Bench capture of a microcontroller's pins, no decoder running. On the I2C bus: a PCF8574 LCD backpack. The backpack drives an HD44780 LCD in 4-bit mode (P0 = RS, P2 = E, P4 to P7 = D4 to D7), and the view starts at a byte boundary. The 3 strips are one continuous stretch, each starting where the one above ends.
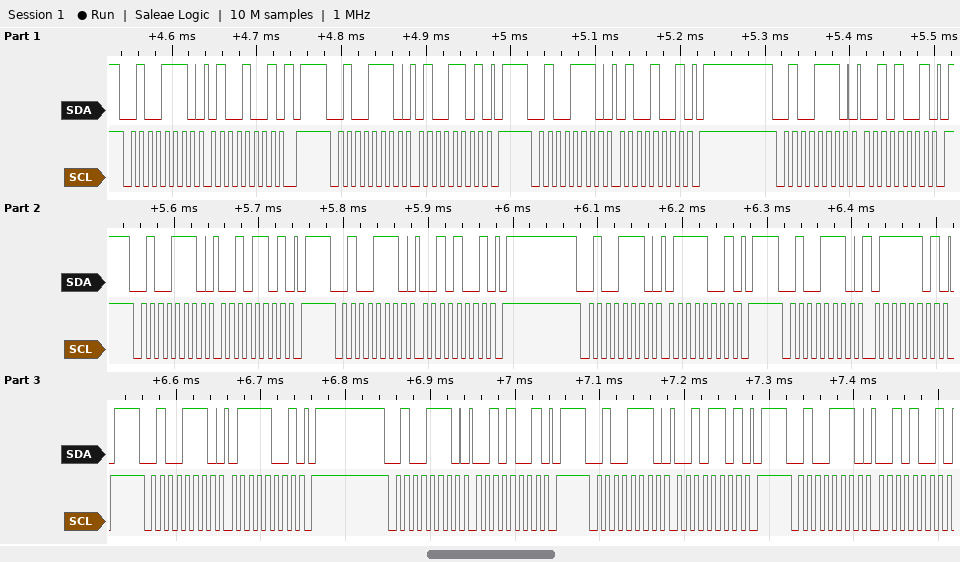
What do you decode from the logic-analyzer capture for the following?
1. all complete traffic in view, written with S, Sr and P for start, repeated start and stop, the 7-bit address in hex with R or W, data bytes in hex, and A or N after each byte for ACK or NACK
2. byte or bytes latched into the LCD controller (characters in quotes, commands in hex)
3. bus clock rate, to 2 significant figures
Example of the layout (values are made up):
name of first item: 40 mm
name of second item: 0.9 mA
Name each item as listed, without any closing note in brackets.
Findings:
all complete traffic in view, written with S, Sr and P for start, repeated start and stop, the 7-bit address in hex with R or W, data bytes in hex, and A or N after each byte for ACK or NACK: S 27W A 49 A P S 27W A 4D A P S 27W A 49 A P S 27W A 29 A P S 27W A 2D A P S 27W A 29 A P S 27W A 79 A P S 27W A 7D A P S 27W A 79 A P S 27W A 29 A P S 27W A 2D A P S 27W A 29 A
byte or bytes latched into the LCD controller: 'B' 'r'
bus clock rate, to 2 significant figures: 100 kHz
